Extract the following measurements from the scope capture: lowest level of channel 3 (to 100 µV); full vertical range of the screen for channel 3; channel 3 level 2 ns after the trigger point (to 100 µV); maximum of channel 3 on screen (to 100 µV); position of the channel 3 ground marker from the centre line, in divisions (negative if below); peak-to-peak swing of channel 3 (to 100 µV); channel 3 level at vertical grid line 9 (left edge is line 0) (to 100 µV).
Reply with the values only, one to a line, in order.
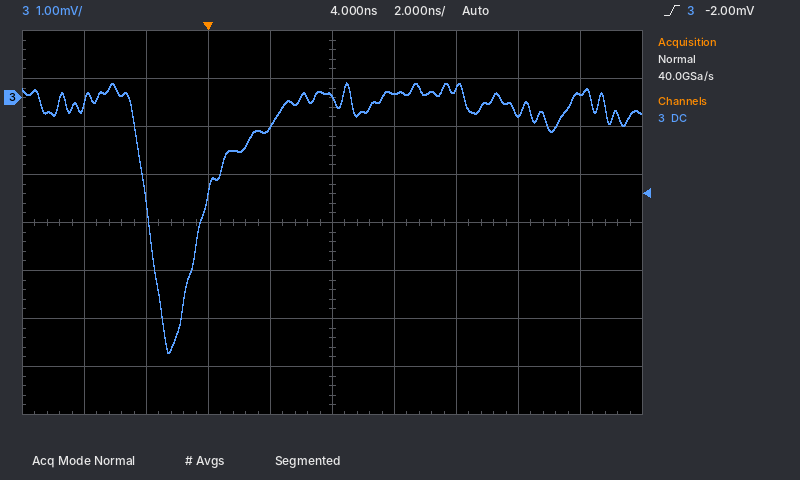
-5.3 mV
8 mV
-600 µV
300 µV
+2.6 div
5.6 mV
100 µV
